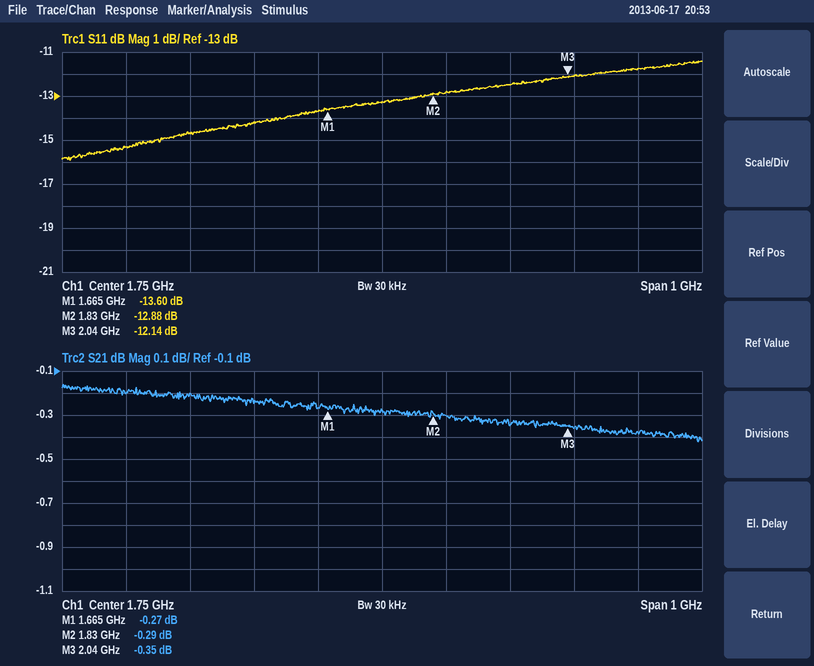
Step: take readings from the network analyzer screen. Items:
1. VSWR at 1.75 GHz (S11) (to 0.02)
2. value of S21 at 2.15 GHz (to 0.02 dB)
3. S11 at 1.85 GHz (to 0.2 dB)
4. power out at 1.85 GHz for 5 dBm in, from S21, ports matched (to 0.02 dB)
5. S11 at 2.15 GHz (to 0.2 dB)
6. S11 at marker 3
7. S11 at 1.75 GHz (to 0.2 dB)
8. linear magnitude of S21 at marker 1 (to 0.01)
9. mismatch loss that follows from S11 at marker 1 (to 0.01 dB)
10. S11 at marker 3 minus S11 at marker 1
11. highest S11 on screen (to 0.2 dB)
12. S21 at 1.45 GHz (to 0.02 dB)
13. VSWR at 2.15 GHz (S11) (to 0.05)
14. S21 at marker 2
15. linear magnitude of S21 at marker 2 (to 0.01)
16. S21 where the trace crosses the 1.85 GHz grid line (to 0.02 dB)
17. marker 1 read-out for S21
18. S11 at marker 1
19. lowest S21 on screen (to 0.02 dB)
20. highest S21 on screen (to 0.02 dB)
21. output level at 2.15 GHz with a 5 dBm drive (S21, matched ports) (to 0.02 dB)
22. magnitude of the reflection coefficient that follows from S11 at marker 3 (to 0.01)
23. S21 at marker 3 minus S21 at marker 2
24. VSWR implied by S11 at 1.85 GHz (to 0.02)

1.56
-0.38 dB
-12.8 dB
4.70 dBm
-11.8 dB
-12.14 dB
-13.2 dB
0.97
0.19 dB
1.46 dB
-11.4 dB
-0.20 dB
1.70
-0.29 dB
0.97
-0.30 dB
-0.27 dB
-13.60 dB
-0.42 dB
-0.16 dB
4.62 dBm
0.25
-0.06 dB
1.60
